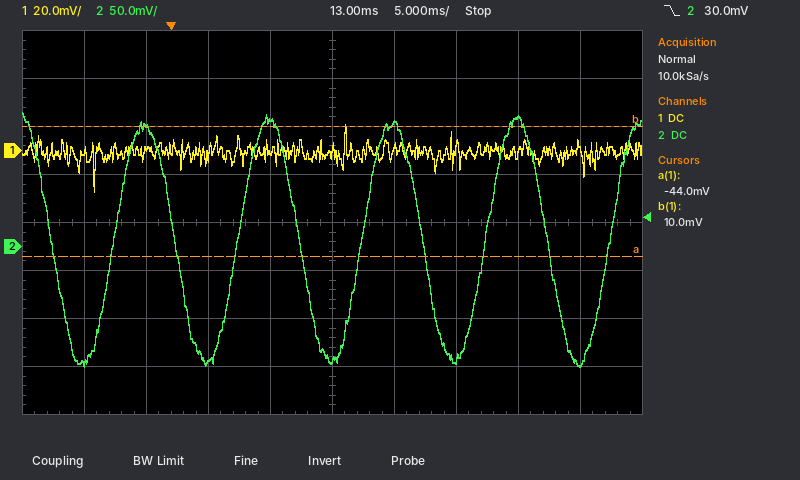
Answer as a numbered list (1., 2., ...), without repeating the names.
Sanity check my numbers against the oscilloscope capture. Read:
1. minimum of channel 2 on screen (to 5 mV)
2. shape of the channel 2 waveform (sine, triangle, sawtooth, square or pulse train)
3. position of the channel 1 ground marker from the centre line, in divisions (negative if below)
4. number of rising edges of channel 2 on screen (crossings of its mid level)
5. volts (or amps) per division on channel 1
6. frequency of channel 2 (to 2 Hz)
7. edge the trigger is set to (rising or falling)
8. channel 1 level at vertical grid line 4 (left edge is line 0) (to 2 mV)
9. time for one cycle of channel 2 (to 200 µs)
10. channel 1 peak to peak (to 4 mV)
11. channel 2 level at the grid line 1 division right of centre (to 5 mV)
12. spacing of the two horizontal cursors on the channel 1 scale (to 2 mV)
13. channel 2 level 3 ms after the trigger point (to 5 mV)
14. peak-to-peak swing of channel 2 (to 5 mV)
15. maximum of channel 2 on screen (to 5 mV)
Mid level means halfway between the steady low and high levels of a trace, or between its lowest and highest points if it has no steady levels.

1. -125 mV
2. sine
3. +1.5 div
4. 5
5. 20 mV
6. 100 Hz
7. falling
8. 0 mV
9. 10.0 ms
10. 28 mV
11. 130 mV
12. 54 mV
13. -120 mV
14. 265 mV
15. 140 mV
